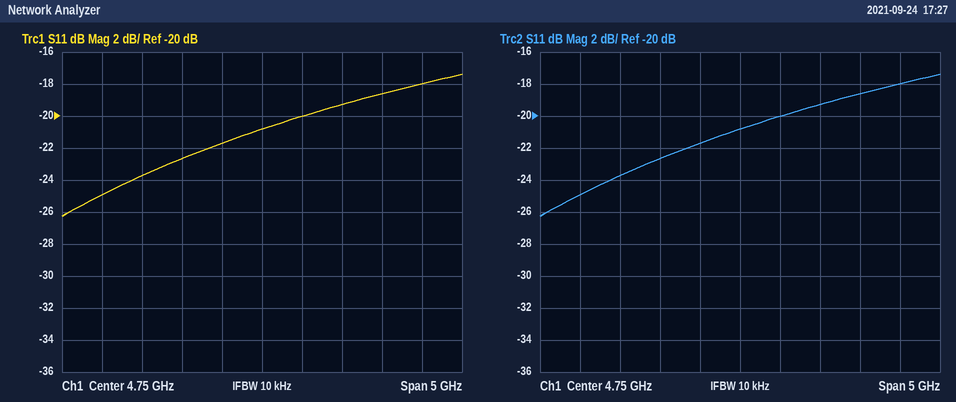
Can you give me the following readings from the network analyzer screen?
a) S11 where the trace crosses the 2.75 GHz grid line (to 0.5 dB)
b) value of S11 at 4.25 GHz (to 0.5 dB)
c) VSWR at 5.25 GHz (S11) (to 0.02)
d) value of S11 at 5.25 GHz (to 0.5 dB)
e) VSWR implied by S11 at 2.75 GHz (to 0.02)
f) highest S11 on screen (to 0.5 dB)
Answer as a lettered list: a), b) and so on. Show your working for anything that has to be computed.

a) -25.0 dB
b) -21.5 dB
c) |Γ| = 10^(-20/20) = 0.1000; VSWR = (1 + 0.1000)/(1 − 0.1000) ≈ 1.22
d) -20.0 dB
e) |Γ| = 10^(-25/20) = 0.0562; VSWR = (1 + 0.0562)/(1 − 0.0562) ≈ 1.12
f) -17.5 dB
